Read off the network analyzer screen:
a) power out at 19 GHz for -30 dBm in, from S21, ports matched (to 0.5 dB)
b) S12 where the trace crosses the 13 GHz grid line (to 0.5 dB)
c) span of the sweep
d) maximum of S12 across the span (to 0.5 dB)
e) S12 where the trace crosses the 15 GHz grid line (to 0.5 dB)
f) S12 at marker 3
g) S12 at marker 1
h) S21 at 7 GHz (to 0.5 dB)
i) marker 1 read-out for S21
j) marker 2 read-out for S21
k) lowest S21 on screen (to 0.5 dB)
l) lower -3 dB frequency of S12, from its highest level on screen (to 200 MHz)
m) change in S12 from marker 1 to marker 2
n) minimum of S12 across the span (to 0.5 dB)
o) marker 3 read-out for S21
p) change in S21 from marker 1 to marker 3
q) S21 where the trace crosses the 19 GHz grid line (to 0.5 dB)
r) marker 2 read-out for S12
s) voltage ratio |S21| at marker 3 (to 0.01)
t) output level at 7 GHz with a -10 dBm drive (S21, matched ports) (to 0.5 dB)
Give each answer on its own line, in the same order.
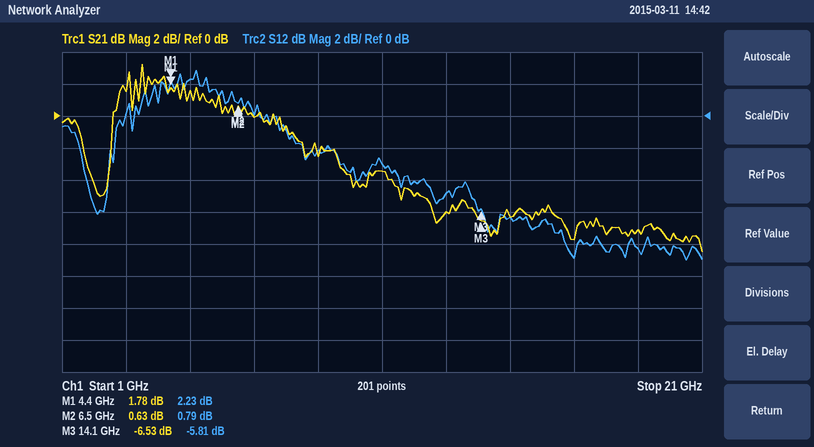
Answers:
-37.0 dBm
-5.0 dB
20 GHz
3.0 dB
-6.5 dB
-5.81 dB
2.23 dB
0.0 dB
1.78 dB
0.63 dB
-8.5 dB
3.2 GHz
-1.44 dB
-9.0 dB
-6.53 dB
-8.31 dB
-7.0 dB
0.79 dB
0.47
-10.0 dBm
